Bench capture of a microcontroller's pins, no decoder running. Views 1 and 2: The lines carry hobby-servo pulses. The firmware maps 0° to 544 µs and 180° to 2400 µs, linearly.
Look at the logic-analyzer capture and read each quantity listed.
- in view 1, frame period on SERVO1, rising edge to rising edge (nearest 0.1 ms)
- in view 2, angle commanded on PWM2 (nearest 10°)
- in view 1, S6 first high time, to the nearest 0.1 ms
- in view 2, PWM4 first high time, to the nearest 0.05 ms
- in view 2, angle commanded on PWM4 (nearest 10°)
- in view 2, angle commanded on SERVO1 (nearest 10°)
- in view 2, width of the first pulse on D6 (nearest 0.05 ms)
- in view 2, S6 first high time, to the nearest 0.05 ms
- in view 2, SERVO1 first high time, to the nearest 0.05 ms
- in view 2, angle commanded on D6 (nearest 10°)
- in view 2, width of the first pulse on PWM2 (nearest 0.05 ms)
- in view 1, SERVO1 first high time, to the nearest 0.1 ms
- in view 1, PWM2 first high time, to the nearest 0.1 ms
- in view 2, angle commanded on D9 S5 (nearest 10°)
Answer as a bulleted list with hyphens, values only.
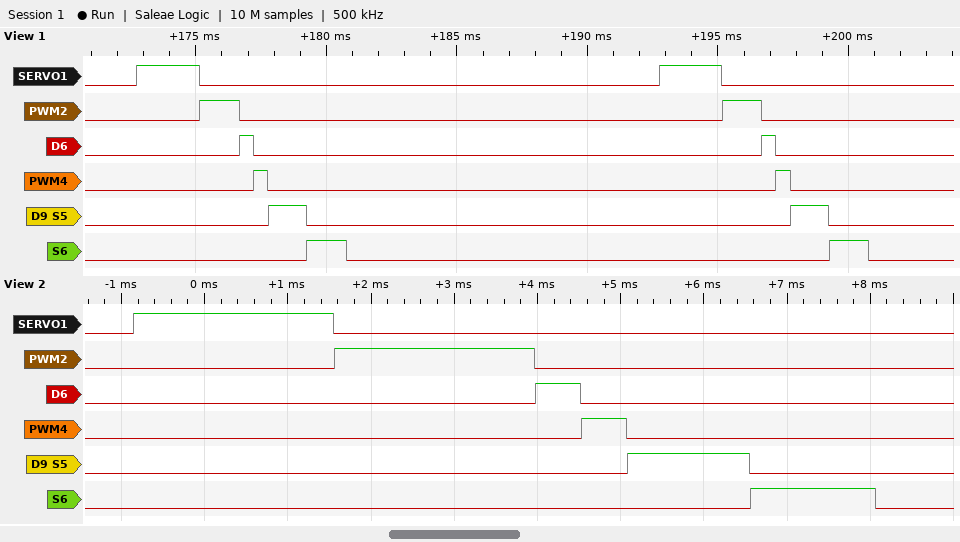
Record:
- 20.0 ms
- 180°
- 1.5 ms
- 0.55 ms
- 0°
- 180°
- 0.55 ms
- 1.50 ms
- 2.40 ms
- 0°
- 2.40 ms
- 2.4 ms
- 1.5 ms
- 90°
